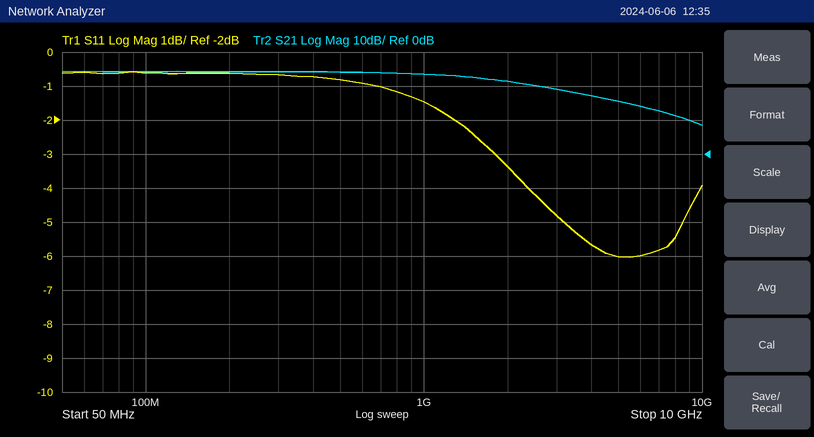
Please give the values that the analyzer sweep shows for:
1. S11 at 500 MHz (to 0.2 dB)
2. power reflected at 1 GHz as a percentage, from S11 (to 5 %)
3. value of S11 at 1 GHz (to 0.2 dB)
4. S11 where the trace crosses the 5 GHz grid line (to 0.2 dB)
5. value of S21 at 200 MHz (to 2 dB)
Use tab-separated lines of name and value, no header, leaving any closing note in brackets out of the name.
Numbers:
S11 at 500 MHz	-0.8 dB
power reflected at 1 GHz as a percentage, from S11	70 %
value of S11 at 1 GHz	-1.4 dB
S11 where the trace crosses the 5 GHz grid line	-6.0 dB
value of S21 at 200 MHz	24 dB
